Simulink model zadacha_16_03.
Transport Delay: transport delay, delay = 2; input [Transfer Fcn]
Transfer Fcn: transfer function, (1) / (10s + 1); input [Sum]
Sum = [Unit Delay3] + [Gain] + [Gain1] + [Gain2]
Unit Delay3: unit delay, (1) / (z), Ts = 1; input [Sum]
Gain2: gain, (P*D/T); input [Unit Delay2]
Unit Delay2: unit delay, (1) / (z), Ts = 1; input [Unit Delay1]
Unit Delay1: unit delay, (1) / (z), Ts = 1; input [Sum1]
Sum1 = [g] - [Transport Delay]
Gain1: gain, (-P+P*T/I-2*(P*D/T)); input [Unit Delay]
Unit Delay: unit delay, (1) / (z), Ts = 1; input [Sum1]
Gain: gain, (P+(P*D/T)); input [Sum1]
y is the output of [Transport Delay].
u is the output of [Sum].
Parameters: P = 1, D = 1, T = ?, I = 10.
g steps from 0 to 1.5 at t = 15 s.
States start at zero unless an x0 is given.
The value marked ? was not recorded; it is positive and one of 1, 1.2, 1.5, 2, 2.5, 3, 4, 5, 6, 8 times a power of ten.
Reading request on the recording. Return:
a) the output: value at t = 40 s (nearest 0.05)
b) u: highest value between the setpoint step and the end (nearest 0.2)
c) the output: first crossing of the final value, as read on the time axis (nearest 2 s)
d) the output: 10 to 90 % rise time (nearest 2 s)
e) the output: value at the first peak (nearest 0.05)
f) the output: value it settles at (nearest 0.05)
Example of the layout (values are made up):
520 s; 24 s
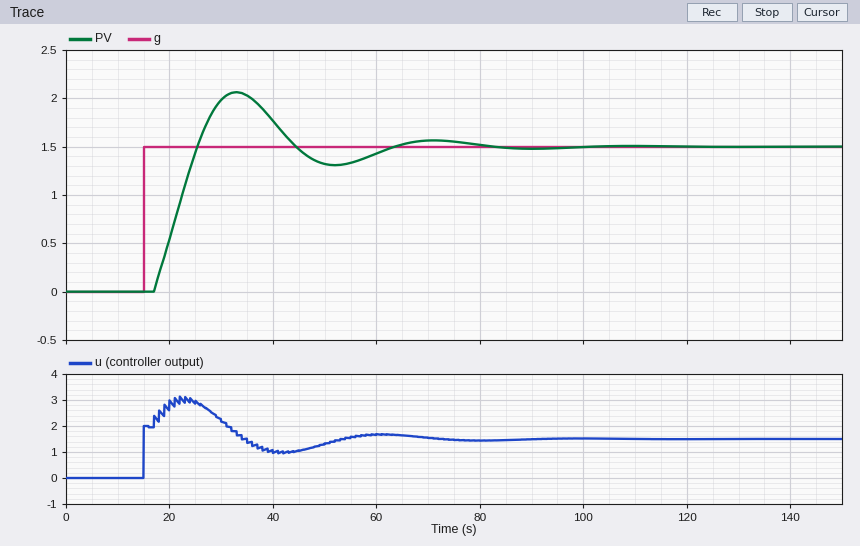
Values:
1.75; 3.2; 26 s; 6 s; 2.05; 1.50
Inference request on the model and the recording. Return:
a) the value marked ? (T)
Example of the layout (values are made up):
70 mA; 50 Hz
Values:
3
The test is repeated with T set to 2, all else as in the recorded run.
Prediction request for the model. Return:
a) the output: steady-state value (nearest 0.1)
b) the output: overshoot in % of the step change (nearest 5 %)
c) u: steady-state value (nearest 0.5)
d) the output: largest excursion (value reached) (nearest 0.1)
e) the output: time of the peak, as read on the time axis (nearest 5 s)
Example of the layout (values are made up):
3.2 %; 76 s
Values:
1.5; 20 %; 1.5; 1.8; 35 s
